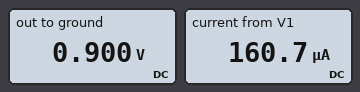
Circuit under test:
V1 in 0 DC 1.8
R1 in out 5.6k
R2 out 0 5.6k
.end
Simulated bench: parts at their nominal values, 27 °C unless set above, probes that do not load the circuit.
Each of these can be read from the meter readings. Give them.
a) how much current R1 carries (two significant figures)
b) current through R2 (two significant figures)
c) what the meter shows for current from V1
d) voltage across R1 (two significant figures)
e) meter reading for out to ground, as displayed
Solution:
160 µA
160 µA
160.7 µA
900 mV
0.900 V
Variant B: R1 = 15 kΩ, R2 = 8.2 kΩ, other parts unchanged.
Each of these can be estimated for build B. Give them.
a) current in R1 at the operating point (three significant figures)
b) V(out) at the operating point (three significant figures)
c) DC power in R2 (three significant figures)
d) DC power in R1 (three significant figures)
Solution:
77.6 µA
636 mV
49.4 µW
90.3 µW
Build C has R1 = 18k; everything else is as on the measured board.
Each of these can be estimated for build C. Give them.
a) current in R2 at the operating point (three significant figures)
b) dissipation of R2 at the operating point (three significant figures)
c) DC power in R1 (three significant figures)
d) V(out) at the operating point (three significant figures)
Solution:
76.3 µA
32.6 µW
105 µW
427 mV
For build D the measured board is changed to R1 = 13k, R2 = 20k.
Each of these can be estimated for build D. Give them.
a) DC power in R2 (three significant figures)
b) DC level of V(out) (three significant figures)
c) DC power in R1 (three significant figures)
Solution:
59.5 µW
1.09 V
38.7 µW
